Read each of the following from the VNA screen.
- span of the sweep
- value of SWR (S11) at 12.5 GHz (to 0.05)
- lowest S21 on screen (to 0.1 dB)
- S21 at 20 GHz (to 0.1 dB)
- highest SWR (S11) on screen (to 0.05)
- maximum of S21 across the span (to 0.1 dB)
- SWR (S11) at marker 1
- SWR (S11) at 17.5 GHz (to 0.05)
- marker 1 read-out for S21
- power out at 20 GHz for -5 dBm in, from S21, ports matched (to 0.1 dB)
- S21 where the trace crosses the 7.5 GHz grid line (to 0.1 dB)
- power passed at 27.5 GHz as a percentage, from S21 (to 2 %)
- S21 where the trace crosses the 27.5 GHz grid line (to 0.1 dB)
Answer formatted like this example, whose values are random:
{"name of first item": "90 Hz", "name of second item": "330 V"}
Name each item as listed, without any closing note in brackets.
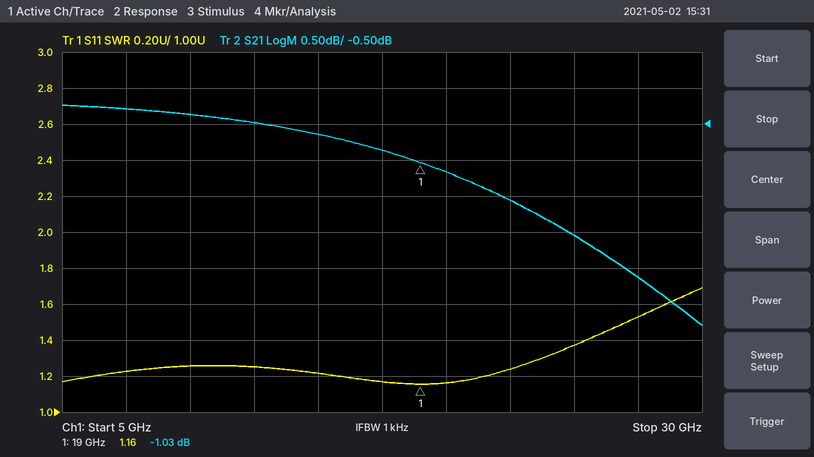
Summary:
{"span of the sweep": "25 GHz", "value of SWR (S11) at 12.5 GHz": "1.25", "lowest S21 on screen": "-3.3 dB", "S21 at 20 GHz": "-1.2 dB", "highest SWR (S11) on screen": "1.70", "maximum of S21 across the span": "-0.2 dB", "SWR (S11) at marker 1": "1.16", "SWR (S11) at 17.5 GHz": "1.15", "marker 1 read-out for S21": "-1.03 dB", "power out at 20 GHz for -5 dBm in, from S21, ports matched": "-6.2 dBm", "S21 where the trace crosses the 7.5 GHz grid line": "-0.3 dB", "power passed at 27.5 GHz as a percentage, from S21": "54 %", "S21 where the trace crosses the 27.5 GHz grid line": "-2.6 dB"}
